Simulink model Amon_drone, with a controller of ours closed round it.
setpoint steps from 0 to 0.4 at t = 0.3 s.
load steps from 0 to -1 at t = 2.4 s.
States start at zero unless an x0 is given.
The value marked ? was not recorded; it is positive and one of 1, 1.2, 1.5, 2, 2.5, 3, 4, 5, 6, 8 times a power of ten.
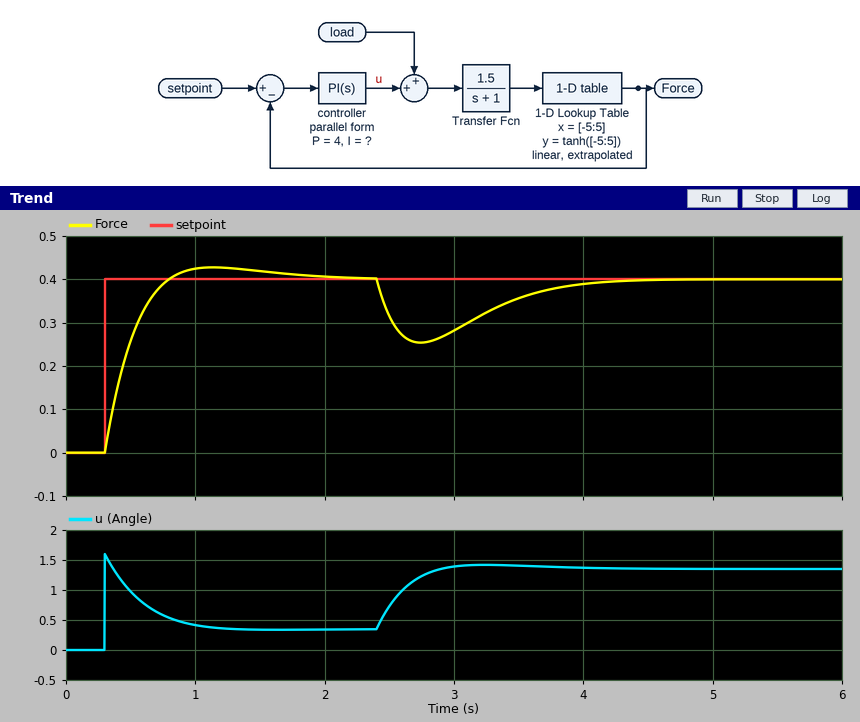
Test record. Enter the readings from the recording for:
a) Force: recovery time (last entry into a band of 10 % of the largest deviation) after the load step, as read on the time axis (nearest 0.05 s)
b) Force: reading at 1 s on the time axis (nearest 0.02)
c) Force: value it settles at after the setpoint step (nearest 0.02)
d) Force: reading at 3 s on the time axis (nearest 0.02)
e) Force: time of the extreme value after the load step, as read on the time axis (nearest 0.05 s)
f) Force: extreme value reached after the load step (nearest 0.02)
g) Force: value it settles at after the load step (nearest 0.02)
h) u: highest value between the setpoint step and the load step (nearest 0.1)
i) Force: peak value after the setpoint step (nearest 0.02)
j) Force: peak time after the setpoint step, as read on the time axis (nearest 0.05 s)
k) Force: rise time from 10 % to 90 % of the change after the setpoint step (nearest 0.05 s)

3.90 s
0.42
0.40
0.28
2.75 s
0.26
0.40
1.6
0.42
1.15 s
0.35 s
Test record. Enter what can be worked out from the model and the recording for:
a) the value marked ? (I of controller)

8
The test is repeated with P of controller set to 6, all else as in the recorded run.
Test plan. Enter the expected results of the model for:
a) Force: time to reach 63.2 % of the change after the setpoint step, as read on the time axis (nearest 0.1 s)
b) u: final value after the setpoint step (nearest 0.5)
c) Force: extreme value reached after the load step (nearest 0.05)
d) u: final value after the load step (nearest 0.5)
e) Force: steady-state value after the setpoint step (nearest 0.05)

0.4 s
0.5
0.30
1.5
0.40
